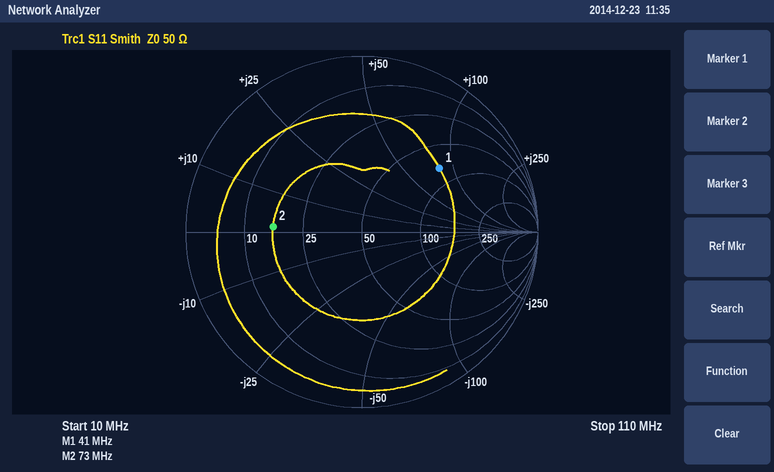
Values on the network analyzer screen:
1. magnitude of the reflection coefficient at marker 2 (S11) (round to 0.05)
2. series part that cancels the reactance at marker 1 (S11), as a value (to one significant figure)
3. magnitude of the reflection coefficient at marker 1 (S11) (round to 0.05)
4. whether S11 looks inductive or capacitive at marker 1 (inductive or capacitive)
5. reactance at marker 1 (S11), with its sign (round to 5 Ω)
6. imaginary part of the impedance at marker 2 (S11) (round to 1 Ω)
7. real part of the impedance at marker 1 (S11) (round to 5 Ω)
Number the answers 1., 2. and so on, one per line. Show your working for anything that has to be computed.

1. 0.50
2. C = 1/(2π × 41 MHz × 80 Ω) ≈ 48.5 pF, so 50 pF to one significant figure
3. 0.55
4. inductive
5. +80 Ω
6. +1 Ω
7. 75 Ω
